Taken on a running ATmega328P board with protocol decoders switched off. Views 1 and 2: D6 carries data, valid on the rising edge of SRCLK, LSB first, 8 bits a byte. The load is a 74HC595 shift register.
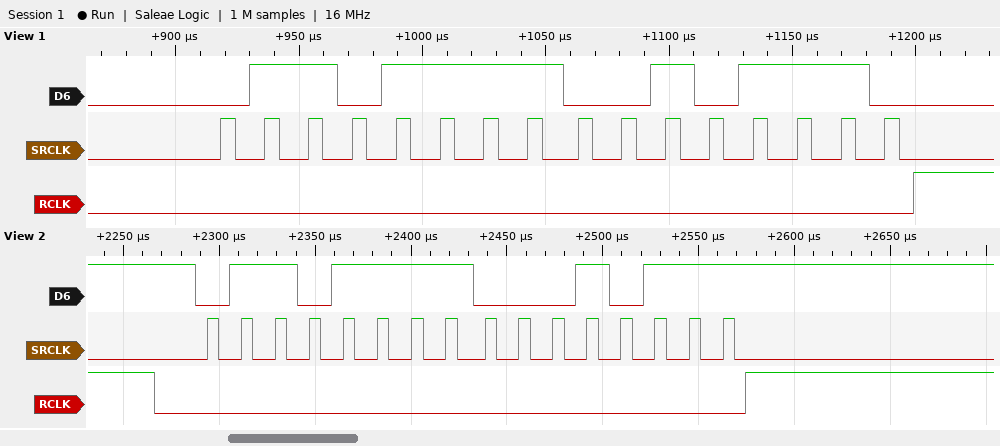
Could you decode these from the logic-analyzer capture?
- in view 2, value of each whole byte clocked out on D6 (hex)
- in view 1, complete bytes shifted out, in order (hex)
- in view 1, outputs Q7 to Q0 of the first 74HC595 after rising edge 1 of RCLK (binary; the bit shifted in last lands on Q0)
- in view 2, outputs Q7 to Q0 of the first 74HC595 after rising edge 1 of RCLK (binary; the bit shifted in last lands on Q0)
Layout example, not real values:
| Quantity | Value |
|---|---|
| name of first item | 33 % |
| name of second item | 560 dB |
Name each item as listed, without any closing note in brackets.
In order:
| Quantity | Value |
|---|---|
| in view 2, value of each whole byte clocked out on D6 | 0xF6 0xE8 |
| in view 1, complete bytes shifted out, in order | 0xF6 0x74 |
| in view 1, outputs Q7 to Q0 of the first 74HC595 after rising edge 1 of RCLK | 00101110 |
| in view 2, outputs Q7 to Q0 of the first 74HC595 after rising edge 1 of RCLK | 00010111 |
